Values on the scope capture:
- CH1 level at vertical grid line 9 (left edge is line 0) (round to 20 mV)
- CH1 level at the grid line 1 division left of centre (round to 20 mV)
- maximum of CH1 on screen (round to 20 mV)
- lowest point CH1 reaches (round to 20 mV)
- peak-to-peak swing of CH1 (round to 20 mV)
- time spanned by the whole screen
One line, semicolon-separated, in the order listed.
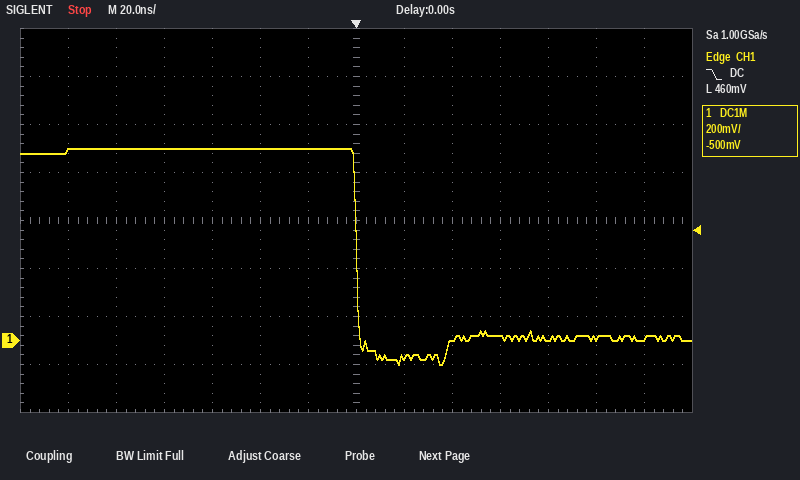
0 mV; 800 mV; 800 mV; -100 mV; 900 mV; 280 ns
